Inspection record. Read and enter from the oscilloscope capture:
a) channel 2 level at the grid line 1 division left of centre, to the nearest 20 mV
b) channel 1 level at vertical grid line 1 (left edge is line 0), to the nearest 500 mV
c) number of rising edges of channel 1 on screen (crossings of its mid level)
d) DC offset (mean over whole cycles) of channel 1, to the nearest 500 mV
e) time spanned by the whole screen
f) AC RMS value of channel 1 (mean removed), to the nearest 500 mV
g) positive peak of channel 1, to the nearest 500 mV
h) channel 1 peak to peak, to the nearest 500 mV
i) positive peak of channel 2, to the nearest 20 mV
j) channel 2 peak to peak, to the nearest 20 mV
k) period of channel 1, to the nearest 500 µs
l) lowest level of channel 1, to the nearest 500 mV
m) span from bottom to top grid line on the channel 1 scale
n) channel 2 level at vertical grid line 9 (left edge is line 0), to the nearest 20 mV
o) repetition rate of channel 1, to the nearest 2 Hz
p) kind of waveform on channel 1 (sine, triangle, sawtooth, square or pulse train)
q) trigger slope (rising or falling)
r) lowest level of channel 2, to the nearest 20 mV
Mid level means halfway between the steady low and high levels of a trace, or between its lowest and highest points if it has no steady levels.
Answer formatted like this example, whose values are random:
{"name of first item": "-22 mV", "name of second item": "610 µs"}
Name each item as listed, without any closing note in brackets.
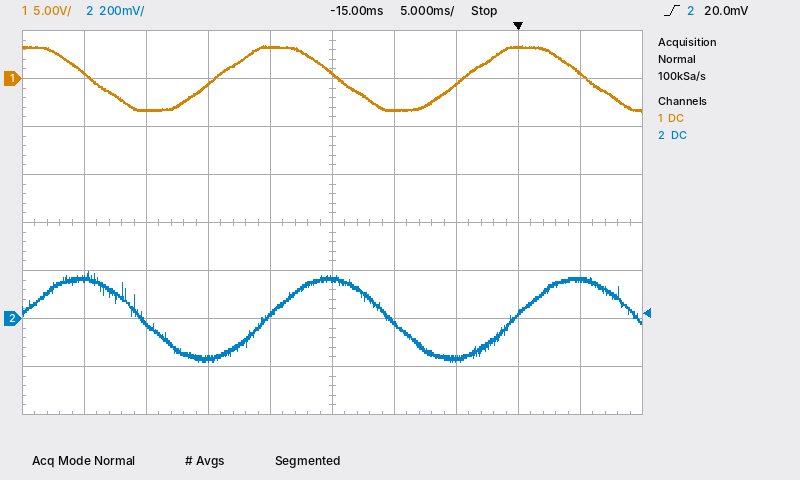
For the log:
{"channel 2 level at the grid line 1 division left of centre, to the nearest 20 mV": "20 mV", "channel 1 level at vertical grid line 1 (left edge is line 0), to the nearest 500 mV": "500 mV", "number of rising edges of channel 1 on screen": "2", "DC offset (mean over whole cycles) of channel 1, to the nearest 500 mV": "0.0 V", "time spanned by the whole screen": "50 ms", "AC RMS value of channel 1 (mean removed), to the nearest 500 mV": "2.5 V", "positive peak of channel 1, to the nearest 500 mV": "3.5 V", "channel 1 peak to peak, to the nearest 500 mV": "7.0 V", "positive peak of channel 2, to the nearest 20 mV": "200 mV", "channel 2 peak to peak, to the nearest 20 mV": "380 mV", "period of channel 1, to the nearest 500 µs": "20.0 ms", "lowest level of channel 1, to the nearest 500 mV": "-3.5 V", "span from bottom to top grid line on the channel 1 scale": "40 V", "channel 2 level at vertical grid line 9 (left edge is line 0), to the nearest 20 mV": "160 mV", "repetition rate of channel 1, to the nearest 2 Hz": "50 Hz", "kind of waveform on channel 1": "sine", "trigger slope": "rising", "lowest level of channel 2, to the nearest 20 mV": "-180 mV"}
